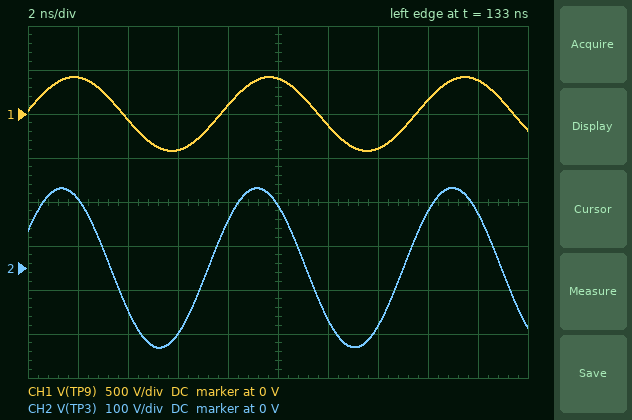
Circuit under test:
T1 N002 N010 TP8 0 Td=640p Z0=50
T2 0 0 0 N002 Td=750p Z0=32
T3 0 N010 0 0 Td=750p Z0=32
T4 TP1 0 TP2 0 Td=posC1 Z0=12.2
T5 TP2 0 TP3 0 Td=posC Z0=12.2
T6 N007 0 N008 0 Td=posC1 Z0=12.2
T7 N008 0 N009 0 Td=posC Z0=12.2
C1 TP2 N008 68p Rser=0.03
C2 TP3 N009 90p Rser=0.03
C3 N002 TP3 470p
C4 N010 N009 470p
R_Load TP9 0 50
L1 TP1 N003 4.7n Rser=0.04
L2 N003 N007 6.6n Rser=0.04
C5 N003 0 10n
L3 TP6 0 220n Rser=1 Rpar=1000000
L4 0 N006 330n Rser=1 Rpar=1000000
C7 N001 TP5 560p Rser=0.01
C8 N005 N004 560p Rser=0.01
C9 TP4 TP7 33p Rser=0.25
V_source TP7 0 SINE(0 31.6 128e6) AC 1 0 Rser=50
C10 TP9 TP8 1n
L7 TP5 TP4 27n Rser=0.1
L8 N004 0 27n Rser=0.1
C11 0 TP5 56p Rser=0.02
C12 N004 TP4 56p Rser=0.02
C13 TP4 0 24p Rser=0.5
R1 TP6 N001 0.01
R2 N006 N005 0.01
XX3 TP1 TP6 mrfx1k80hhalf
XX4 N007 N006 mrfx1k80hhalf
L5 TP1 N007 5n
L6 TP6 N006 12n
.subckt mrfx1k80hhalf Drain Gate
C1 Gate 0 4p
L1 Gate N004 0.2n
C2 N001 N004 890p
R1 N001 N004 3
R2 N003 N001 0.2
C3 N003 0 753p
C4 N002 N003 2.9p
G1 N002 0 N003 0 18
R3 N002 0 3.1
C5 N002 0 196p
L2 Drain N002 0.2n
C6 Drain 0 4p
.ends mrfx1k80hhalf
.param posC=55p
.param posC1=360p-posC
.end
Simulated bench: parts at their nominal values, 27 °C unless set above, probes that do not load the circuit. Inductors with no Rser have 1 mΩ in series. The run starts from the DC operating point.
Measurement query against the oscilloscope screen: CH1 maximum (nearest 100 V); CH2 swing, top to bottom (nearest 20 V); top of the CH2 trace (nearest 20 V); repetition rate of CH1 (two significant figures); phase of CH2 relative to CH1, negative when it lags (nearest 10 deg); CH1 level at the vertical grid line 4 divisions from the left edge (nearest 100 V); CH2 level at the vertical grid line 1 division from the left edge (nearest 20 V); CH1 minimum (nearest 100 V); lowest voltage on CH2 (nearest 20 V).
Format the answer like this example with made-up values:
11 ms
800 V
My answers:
400 V
360 V
180 V
130 MHz
20 deg
100 V
160 V
-400 V
-180 V
